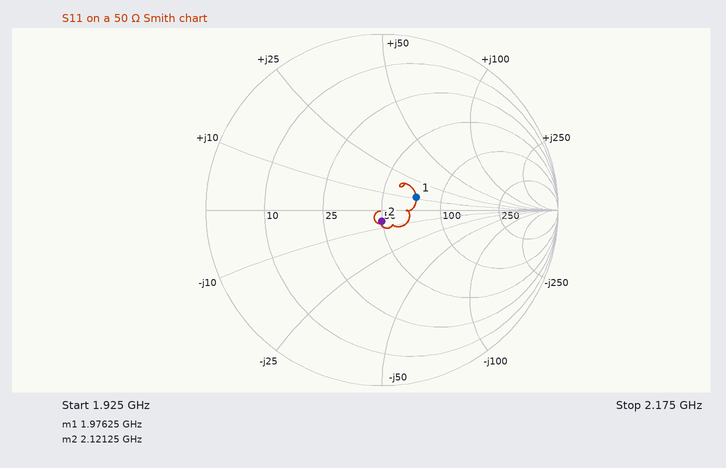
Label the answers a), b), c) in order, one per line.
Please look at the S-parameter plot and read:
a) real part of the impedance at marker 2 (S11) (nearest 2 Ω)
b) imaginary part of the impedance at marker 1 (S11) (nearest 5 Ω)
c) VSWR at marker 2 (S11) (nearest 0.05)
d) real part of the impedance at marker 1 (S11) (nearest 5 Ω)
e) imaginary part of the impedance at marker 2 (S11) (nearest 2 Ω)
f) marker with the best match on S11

a) 50 Ω
b) +10 Ω
c) 1.15
d) 75 Ω
e) -6 Ω
f) marker 2
